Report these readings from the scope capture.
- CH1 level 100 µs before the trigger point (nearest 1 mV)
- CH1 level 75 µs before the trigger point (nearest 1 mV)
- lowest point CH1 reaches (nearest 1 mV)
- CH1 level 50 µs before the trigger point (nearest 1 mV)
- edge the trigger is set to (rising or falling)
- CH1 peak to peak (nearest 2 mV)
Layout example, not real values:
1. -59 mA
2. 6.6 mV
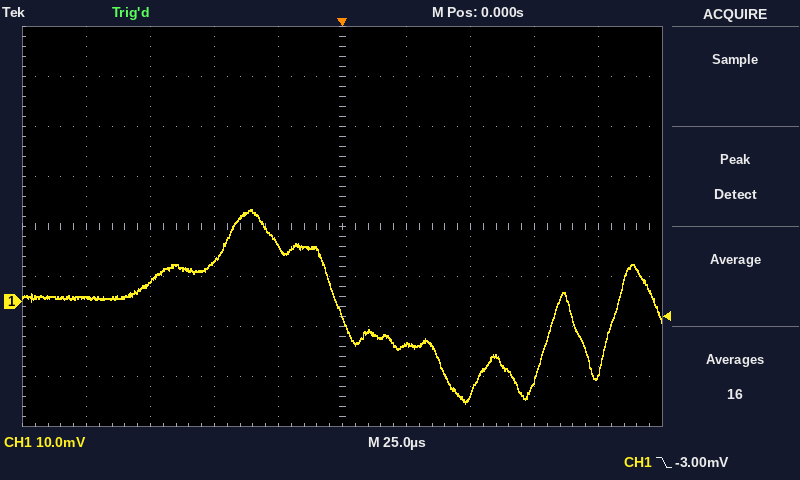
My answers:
1. 1 mV
2. 4 mV
3. -20 mV
4. 8 mV
5. falling
6. 38 mV
